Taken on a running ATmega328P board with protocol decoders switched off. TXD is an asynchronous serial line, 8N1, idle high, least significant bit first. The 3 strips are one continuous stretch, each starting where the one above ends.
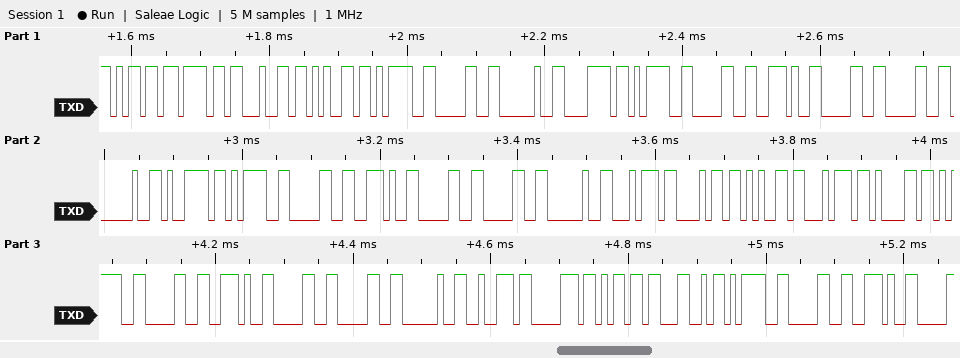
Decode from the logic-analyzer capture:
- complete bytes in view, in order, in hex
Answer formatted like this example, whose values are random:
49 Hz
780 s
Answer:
6D 6F 64 65 3D 30 20 78 3D 30 2E 30 30 20 79 3D 30 2E 30 30 20 74 68 65 74 61 3D 30 2E 30 30 20 72 70 6D 4C 3D 30 2E
